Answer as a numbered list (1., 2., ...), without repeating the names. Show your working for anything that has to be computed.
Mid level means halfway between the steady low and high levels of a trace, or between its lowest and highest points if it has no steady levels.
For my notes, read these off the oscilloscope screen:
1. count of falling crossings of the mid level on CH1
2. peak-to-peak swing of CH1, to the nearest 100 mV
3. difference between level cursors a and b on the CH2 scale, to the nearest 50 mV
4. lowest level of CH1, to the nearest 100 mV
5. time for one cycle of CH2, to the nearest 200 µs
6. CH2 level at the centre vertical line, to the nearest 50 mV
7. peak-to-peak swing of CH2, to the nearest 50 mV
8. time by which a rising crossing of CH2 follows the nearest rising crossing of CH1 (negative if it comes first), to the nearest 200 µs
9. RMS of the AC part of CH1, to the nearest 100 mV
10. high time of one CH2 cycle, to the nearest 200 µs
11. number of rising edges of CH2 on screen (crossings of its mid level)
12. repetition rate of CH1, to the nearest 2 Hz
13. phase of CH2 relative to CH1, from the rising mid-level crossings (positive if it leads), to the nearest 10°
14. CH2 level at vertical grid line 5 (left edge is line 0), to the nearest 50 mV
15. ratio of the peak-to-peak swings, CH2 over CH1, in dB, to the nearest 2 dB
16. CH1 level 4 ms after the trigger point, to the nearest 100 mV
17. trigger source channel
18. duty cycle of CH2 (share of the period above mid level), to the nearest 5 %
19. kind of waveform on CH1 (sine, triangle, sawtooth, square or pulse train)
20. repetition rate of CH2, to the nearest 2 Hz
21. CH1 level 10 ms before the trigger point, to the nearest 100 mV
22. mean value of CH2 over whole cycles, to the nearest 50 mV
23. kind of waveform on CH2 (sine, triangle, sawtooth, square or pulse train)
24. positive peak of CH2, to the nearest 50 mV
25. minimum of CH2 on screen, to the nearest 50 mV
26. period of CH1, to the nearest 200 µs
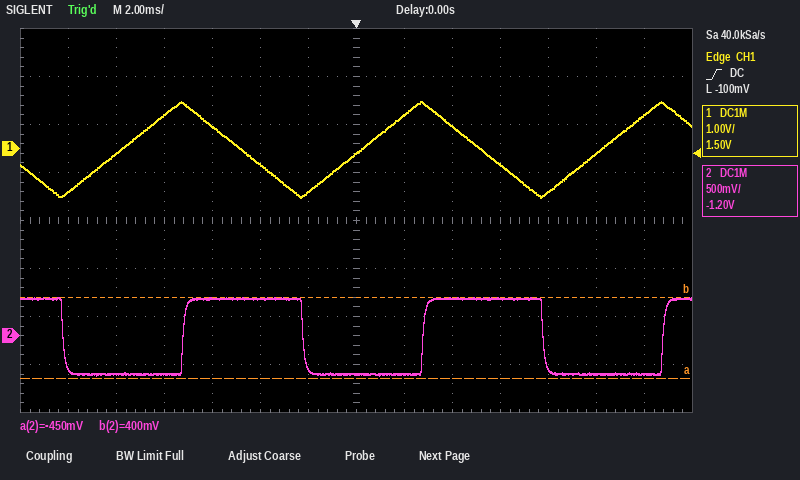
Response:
1. 2
2. 1.0 V − (-1.0 V) = 2.0 V
3. 850 mV
4. -1.0 V
5. 10.0 ms
6. -400 mV
7. 400 mV − (-400 mV) = 800 mV
8. +2.6 ms
9. 2.0 V / (2√3) ≈ 577 mV, so 600 mV to the nearest 100 mV
10. 5.0 ms
11. 3
12. 1 / 10.0 ms ≈ 100 Hz
13. −360° × (+2.6 ms) / 10.0 ms ≈ -93.6°, so -90° to the nearest 10°
14. 400 mV
15. 20 log10(800 mV / 2.0 V) ≈ -8 dB
16. 500 mV
17. CH1
18. 5.0 ms / 10.0 ms ≈ 50 %
19. triangle
20. 1 / 10.0 ms ≈ 100 Hz
21. -100 mV
22. -400 mV + 0.5 × (400 mV − (-400 mV)) ≈ 0 mV
23. square
24. 400 mV
25. -400 mV
26. 10.0 ms
